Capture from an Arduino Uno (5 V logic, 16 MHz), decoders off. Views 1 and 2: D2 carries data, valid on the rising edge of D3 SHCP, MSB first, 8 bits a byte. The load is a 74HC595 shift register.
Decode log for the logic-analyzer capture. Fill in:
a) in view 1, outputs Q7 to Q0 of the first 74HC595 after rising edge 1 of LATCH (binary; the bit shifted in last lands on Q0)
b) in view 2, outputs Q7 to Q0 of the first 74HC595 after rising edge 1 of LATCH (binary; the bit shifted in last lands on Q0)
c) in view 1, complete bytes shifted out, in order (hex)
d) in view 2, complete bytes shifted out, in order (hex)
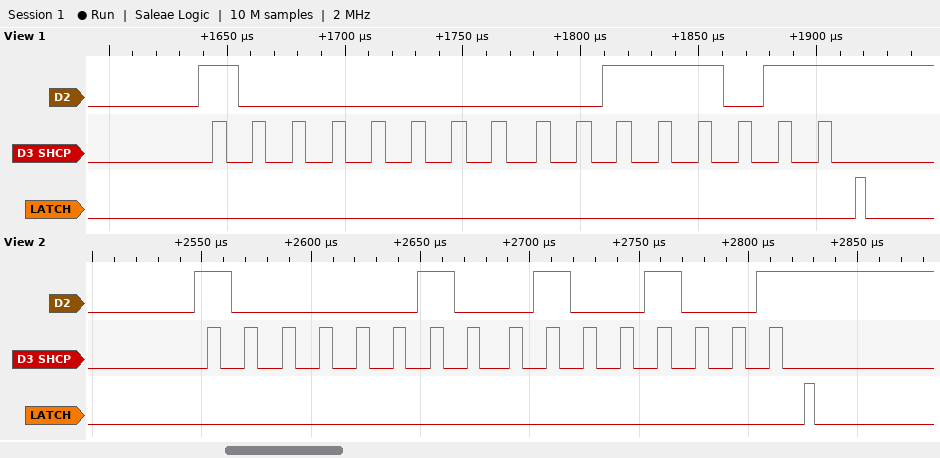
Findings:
00111011
01001001
80 3B
82 49
